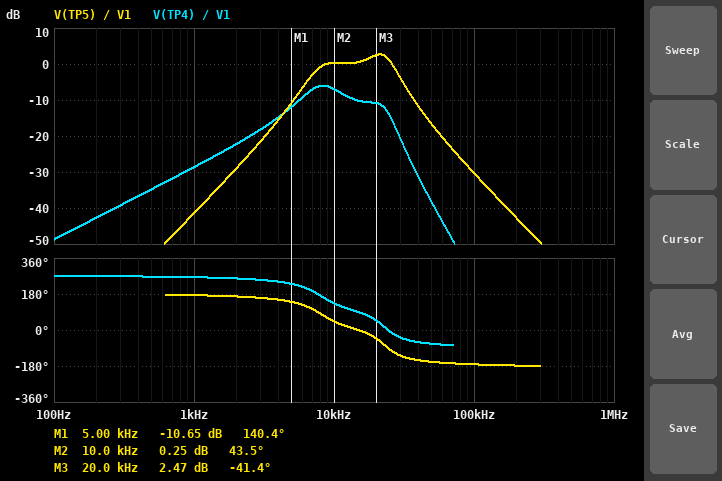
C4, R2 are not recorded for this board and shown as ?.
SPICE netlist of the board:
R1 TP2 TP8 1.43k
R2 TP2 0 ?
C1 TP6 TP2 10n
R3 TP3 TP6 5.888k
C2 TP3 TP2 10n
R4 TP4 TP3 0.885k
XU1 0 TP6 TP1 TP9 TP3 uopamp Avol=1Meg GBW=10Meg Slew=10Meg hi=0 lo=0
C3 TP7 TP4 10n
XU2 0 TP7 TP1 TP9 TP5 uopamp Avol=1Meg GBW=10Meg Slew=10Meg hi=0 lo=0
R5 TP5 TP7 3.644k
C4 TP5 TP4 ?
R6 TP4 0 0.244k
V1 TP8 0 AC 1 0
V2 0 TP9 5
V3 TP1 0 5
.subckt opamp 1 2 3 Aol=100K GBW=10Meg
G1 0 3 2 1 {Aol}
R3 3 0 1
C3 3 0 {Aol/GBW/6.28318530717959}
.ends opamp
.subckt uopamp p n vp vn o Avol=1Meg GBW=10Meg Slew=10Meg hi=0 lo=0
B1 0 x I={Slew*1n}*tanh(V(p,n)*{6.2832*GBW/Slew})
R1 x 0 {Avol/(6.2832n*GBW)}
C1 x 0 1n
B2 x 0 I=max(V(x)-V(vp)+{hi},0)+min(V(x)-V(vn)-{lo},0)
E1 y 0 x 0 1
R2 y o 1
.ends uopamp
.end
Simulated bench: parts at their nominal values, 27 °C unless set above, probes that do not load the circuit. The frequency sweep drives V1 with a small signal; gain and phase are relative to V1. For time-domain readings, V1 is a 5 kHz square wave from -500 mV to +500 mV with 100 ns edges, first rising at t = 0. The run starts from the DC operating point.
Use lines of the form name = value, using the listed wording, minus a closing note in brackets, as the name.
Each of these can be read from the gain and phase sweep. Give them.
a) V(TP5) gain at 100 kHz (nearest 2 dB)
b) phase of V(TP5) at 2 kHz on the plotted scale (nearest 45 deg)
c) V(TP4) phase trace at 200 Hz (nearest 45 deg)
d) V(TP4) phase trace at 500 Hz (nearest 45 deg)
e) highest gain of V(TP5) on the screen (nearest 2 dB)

V(TP5) gain at 100 kHz = -30 dB
phase of V(TP5) at 2 kHz on the plotted scale = 180 deg
V(TP4) phase trace at 200 Hz = 270 deg
V(TP4) phase trace at 500 Hz = 270 deg
highest gain of V(TP5) on the screen = 2 dB
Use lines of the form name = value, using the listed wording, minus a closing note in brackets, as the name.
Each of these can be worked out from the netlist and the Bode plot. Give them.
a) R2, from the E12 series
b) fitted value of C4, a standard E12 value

R2, from the E12 series = 1.2 kΩ
fitted value of C4, a standard E12 value = 6.8 nF
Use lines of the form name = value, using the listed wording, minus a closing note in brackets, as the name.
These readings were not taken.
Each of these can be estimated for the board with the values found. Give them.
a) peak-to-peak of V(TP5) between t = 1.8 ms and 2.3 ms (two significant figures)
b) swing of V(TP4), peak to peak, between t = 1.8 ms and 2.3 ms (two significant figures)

peak-to-peak of V(TP5) between t = 1.8 ms and 2.3 ms = 830 mV
swing of V(TP4), peak to peak, between t = 1.8 ms and 2.3 ms = 490 mV
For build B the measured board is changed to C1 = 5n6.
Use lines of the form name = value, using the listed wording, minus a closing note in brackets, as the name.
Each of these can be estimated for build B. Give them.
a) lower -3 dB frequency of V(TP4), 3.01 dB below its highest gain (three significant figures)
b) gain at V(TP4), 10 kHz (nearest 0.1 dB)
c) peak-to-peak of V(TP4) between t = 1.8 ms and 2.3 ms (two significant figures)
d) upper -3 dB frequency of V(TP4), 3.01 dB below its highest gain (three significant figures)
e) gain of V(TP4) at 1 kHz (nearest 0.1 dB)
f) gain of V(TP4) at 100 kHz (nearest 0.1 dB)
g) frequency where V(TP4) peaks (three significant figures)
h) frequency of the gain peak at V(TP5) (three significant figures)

lower -3 dB frequency of V(TP4), 3.01 dB below its highest gain = 8.28 kHz
gain at V(TP4), 10 kHz = -8.6 dB
peak-to-peak of V(TP4) between t = 1.8 ms and 2.3 ms = 350 mV
upper -3 dB frequency of V(TP4), 3.01 dB below its highest gain = 22.2 kHz
gain of V(TP4) at 1 kHz = -33.7 dB
gain of V(TP4) at 100 kHz = -59.7 dB
frequency where V(TP4) peaks = 11.6 kHz
frequency of the gain peak at V(TP5) = 21.1 kHz
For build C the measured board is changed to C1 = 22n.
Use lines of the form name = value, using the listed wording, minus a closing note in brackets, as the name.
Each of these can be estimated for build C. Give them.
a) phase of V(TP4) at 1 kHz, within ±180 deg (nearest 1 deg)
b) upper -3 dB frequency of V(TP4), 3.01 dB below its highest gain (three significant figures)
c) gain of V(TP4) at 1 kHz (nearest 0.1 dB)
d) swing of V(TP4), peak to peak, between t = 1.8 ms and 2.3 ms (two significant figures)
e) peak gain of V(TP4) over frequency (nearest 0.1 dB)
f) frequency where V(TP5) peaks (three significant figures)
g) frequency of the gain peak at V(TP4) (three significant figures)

phase of V(TP4) at 1 kHz, within ±180 deg = -99 deg
upper -3 dB frequency of V(TP4), 3.01 dB below its highest gain = 8.10 kHz
gain of V(TP4) at 1 kHz = -21.7 dB
swing of V(TP4), peak to peak, between t = 1.8 ms and 2.3 ms = 900 mV
peak gain of V(TP4) over frequency = -3.8 dB
frequency where V(TP5) peaks = 21.6 kHz
frequency of the gain peak at V(TP4) = 5.54 kHz
